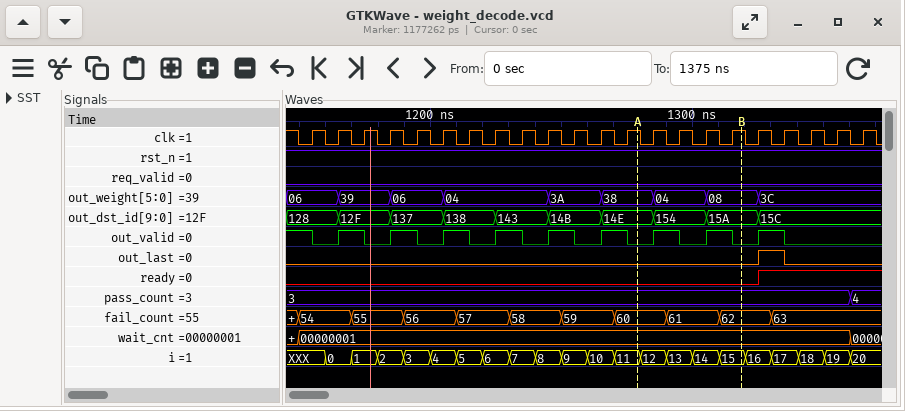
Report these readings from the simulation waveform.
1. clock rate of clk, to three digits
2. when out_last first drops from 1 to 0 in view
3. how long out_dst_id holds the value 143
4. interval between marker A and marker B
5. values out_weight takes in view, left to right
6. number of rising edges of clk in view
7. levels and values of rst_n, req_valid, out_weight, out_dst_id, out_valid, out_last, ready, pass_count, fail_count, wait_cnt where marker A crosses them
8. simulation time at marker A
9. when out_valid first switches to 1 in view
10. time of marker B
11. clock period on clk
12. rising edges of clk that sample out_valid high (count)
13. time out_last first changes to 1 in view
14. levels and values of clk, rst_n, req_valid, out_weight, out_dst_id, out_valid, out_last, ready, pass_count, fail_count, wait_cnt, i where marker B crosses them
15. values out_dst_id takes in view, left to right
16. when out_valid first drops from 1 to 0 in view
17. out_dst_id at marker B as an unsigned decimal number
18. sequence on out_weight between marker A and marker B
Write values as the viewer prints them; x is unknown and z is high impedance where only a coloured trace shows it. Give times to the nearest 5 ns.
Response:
100 MHz
1335 ns
20 ns
40 ns
06, 39, 06, 04, 3A, 38, 04, 08, 3C
22
rst_n=1, req_valid=0, out_weight=38, out_dst_id=14E, out_valid=0, out_last=0, ready=0, pass_count=3, fail_count=60, wait_cnt=00000001
1280 ns
1165 ns
1320 ns
10 ns
10
1325 ns
clk=1, rst_n=1, req_valid=0, out_weight=08, out_dst_id=15A, out_valid=0, out_last=0, ready=0, pass_count=3, fail_count=62, wait_cnt=00000001, i=15
128, 12F, 137, 138, 143, 14B, 14E, 154, 15A, 15C
1155 ns
346
38, 04, 08
